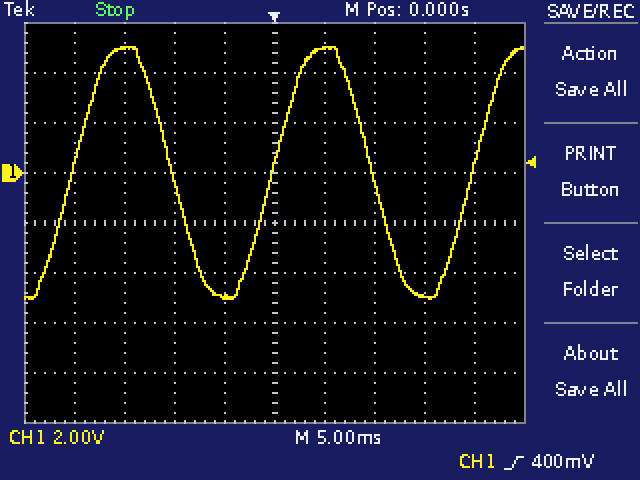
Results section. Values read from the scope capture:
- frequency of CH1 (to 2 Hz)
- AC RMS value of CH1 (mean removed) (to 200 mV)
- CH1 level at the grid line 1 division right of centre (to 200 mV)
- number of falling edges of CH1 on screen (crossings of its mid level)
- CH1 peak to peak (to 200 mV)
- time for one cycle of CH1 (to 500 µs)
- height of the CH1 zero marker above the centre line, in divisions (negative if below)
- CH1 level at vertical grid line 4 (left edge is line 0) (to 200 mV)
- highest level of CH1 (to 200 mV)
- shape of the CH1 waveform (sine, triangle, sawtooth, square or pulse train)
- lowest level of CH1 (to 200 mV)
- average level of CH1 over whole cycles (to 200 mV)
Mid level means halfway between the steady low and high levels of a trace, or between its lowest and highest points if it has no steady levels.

50 Hz
3.6 V
5.0 V
2
10.0 V
20.0 ms
+1.0 div
-5.0 V
5.0 V
sine
-5.0 V
0.0 V
